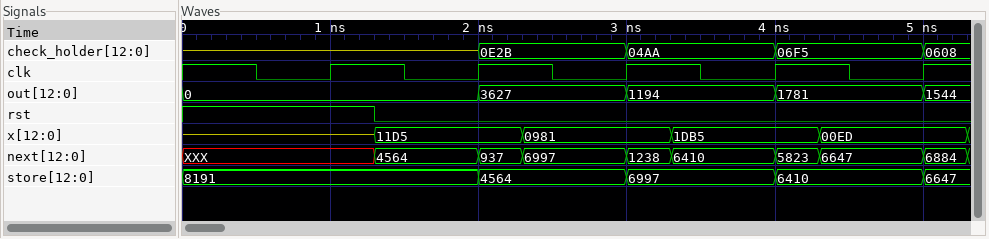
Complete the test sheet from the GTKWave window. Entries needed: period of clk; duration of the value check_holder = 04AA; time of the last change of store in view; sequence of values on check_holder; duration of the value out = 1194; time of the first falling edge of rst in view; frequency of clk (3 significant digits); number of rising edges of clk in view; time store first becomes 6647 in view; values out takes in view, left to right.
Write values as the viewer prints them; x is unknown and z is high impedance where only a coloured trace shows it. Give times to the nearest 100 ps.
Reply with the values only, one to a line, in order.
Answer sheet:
1000 ps
1000 ps
5000 ps
z, 0E2B, 04AA, 06F5, 0608
1000 ps
1300 ps
1.00 GHz
5
5000 ps
0, 3627, 1194, 1781, 1544
